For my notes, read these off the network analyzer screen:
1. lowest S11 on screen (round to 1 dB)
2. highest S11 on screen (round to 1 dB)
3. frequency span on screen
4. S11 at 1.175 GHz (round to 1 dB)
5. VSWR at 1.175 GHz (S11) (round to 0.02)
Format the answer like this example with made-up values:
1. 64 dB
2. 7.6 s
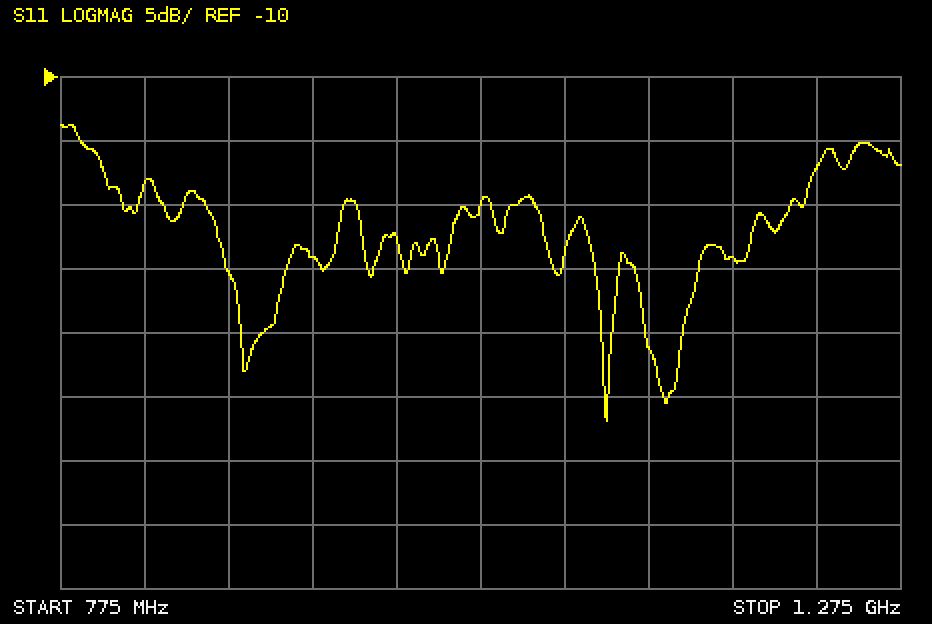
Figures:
1. -37 dB
2. -14 dB
3. 500 MHz
4. -24 dB
5. 1.14
